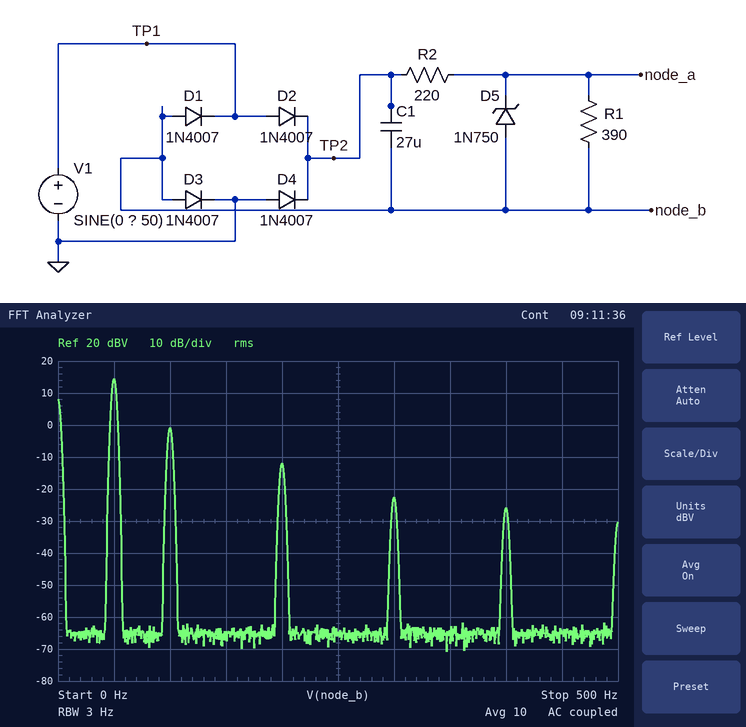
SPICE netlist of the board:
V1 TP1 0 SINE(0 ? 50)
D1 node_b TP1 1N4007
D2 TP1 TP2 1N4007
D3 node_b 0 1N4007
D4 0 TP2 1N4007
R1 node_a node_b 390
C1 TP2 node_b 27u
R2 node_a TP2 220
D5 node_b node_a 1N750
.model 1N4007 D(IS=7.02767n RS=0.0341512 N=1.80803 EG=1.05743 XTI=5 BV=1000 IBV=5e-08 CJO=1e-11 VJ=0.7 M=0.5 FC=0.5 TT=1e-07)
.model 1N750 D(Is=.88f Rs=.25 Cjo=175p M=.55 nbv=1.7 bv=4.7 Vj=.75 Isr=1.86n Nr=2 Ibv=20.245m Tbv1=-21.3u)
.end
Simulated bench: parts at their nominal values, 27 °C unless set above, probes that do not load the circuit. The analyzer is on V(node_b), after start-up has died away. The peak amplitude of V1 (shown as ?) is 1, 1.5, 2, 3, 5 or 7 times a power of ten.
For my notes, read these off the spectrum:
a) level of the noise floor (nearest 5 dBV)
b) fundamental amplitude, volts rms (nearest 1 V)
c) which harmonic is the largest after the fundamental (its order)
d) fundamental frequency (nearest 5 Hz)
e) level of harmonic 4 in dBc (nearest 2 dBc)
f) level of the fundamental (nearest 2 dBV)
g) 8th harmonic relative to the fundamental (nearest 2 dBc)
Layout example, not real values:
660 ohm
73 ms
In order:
-65 dBV
5 V
2
50 Hz
-26 dBc
14 dBV
-40 dBc
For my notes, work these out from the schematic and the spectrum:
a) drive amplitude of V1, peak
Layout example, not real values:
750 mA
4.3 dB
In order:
15 V
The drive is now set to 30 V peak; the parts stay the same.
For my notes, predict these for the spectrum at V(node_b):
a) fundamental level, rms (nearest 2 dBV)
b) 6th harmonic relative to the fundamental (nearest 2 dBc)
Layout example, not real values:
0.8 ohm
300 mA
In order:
20 dBV
-36 dBc
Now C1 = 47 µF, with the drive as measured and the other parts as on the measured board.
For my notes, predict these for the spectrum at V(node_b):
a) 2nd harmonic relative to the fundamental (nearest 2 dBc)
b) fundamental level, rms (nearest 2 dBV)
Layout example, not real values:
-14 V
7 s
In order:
-18 dBc
14 dBV
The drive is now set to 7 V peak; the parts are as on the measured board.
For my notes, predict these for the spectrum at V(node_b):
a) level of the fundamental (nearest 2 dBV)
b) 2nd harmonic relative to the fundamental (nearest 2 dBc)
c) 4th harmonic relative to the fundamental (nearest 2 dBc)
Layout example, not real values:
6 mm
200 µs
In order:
8 dBV
-18 dBc
-28 dBc
